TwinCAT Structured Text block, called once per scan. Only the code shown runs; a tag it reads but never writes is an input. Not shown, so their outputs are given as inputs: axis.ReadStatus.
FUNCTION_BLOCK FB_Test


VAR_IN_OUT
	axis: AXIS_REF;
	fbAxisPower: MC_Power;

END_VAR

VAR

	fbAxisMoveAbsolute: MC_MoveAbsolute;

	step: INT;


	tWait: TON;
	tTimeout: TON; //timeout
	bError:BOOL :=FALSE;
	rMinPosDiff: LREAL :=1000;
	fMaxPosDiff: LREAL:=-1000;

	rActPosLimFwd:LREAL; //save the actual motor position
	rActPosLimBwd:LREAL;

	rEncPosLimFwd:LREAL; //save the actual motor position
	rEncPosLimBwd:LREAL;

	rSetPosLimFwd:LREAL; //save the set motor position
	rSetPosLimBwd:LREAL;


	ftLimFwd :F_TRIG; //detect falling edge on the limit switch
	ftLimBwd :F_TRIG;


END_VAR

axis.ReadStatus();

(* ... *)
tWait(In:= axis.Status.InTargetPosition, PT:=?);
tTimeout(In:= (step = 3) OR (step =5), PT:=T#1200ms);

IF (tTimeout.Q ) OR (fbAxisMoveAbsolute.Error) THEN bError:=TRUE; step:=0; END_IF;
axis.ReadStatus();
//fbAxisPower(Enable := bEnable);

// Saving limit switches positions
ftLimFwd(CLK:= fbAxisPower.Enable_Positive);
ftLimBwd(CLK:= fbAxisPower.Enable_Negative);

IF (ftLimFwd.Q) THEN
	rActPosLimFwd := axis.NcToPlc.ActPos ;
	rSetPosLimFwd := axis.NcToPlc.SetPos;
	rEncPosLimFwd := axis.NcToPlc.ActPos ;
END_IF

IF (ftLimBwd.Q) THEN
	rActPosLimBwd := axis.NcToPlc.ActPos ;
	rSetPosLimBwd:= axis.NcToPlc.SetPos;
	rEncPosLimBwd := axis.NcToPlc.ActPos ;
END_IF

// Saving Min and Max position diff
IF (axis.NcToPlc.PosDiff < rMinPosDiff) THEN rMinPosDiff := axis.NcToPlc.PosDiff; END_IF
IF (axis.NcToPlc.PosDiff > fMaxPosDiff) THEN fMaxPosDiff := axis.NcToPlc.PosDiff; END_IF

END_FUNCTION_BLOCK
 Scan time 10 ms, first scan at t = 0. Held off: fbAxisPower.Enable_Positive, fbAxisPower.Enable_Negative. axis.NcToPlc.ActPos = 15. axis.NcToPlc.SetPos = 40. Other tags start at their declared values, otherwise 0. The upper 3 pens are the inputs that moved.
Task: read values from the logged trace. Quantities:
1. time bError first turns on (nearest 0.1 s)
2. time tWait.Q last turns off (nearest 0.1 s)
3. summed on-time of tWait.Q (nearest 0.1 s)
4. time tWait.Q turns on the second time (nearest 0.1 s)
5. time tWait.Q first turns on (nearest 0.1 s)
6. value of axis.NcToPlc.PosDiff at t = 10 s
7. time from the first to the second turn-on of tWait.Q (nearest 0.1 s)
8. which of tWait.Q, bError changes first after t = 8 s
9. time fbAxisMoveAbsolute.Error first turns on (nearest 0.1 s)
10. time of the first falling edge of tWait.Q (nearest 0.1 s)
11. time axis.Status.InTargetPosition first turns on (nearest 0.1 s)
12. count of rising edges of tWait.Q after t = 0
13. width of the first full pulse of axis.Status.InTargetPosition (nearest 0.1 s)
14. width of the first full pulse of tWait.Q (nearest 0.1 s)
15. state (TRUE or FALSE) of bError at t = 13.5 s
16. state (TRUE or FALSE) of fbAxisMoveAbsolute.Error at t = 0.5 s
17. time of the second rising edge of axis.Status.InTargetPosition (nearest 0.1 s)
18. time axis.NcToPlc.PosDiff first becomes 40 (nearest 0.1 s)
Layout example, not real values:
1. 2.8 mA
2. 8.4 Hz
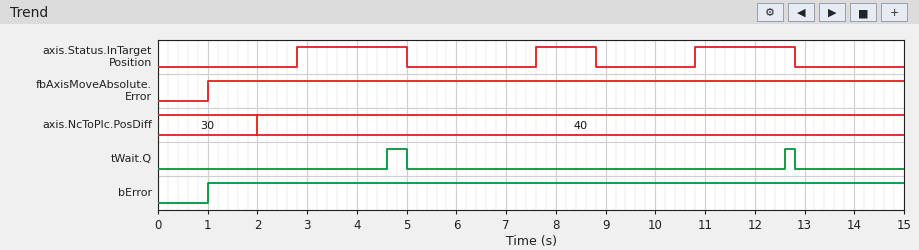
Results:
1. 1.0 s
2. 12.8 s
3. 0.6 s
4. 12.6 s
5. 4.6 s
6. 40
7. 8.0 s
8. tWait.Q
9. 1.0 s
10. 5.0 s
11. 2.8 s
12. 2
13. 2.2 s
14. 0.4 s
15. TRUE
16. FALSE
17. 7.6 s
18. 2.0 s
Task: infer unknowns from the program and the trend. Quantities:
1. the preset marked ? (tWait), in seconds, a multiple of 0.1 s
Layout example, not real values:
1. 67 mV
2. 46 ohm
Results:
1. 1.8 s
